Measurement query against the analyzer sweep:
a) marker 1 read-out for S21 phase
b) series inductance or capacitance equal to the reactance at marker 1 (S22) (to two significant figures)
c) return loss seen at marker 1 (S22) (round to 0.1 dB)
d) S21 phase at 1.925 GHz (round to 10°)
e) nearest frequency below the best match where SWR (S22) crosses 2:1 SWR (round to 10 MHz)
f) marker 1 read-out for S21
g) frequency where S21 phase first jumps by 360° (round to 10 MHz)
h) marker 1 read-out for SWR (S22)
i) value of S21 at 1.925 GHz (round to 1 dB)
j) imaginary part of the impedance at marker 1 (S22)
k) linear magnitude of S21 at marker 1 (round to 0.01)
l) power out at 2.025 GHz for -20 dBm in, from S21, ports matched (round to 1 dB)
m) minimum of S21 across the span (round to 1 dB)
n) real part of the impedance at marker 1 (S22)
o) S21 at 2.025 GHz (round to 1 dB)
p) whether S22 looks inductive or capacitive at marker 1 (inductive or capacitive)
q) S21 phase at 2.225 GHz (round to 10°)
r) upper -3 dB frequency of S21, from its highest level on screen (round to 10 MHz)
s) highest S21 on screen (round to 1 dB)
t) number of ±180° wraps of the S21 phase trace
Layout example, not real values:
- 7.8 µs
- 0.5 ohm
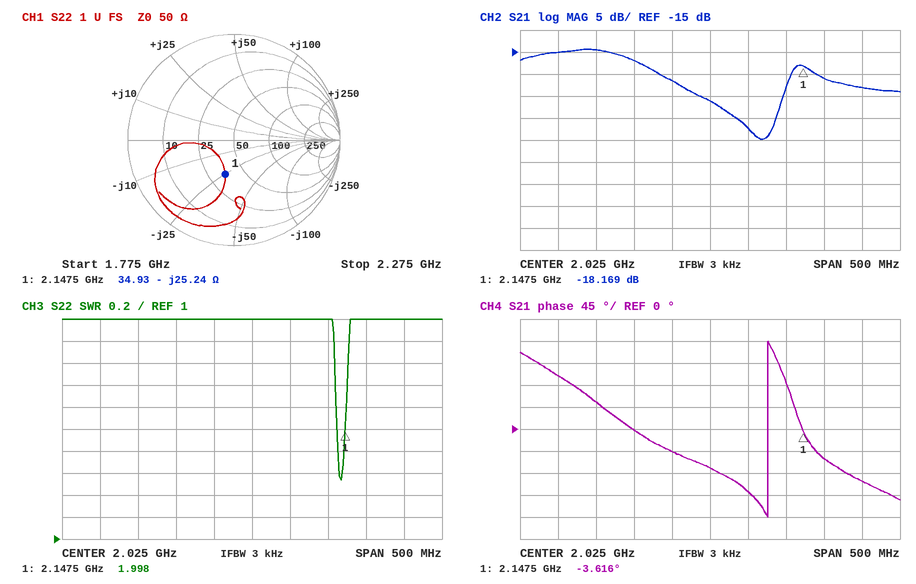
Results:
- -3.616°
- 2.9 pF
- 9.6 dB
- 0°
- 2.14 GHz
- -18.169 dB
- 2.10 GHz
- 1.998
- -17 dB
- -25.24 Ω
- 0.12
- -46 dBm
- -35 dB
- 34.93 Ω
- -26 dB
- capacitive
- -110°
- 1.93 GHz
- -14 dB
- 1
